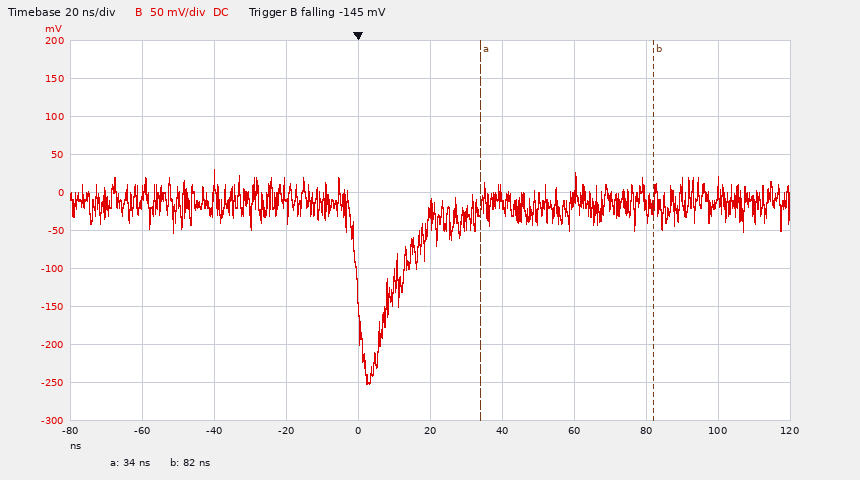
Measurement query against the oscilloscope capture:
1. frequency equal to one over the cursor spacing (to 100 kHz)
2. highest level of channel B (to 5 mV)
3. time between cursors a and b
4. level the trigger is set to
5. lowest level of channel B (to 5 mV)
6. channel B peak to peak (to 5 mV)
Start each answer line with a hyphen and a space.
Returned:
- 20.8 MHz
- 30 mV
- 48 ns
- -145 mV
- -250 mV
- 280 mV
